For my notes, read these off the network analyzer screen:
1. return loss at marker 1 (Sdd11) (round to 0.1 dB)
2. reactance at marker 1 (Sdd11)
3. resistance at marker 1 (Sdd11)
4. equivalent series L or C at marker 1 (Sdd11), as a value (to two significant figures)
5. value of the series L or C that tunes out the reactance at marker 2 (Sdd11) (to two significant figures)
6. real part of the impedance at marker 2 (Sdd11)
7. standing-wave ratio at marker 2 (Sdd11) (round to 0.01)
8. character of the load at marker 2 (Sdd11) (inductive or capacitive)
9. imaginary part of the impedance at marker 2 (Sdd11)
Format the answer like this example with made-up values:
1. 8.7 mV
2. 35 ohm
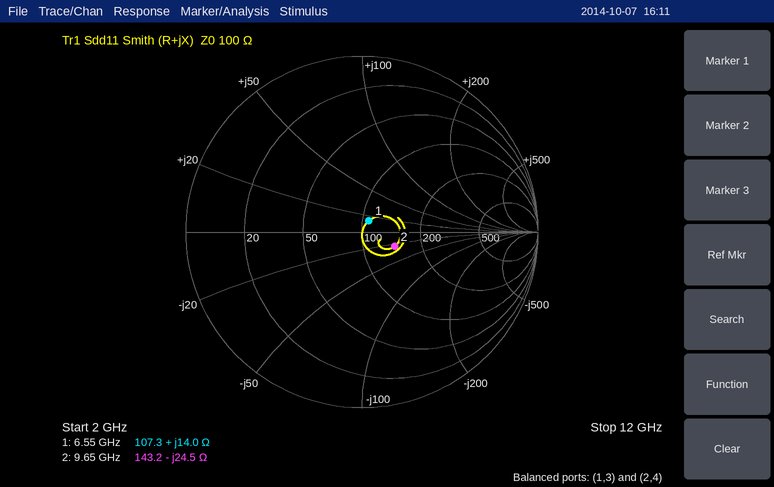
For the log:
1. 22.4 dB
2. +14.0 Ω
3. 107.3 Ω
4. 340 pH
5. 400 pH
6. 143.2 Ω
7. 1.51
8. capacitive
9. -24.5 Ω
